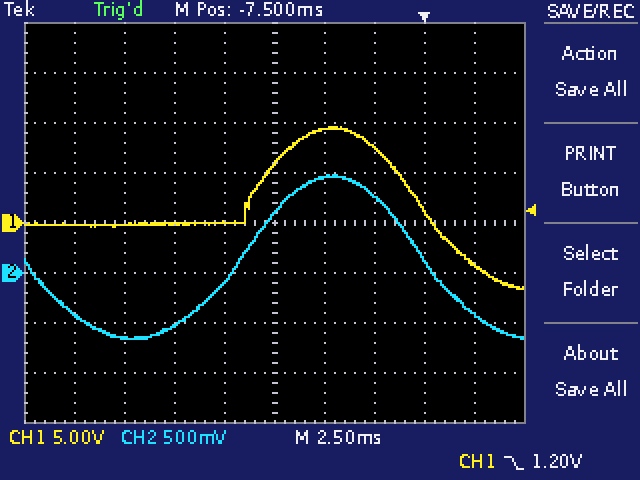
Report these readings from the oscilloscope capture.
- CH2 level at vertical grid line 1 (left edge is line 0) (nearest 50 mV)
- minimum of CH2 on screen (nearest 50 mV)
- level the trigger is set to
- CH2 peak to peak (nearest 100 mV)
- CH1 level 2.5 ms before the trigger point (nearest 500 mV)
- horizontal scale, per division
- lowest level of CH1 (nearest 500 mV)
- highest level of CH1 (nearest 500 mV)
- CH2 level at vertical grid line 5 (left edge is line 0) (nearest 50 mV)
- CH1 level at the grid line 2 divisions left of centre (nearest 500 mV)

-400 mV
-650 mV
1.20 V
1.60 V
7.5 V
2.5 ms
-6.5 V
9.5 V
600 mV
0.0 V
